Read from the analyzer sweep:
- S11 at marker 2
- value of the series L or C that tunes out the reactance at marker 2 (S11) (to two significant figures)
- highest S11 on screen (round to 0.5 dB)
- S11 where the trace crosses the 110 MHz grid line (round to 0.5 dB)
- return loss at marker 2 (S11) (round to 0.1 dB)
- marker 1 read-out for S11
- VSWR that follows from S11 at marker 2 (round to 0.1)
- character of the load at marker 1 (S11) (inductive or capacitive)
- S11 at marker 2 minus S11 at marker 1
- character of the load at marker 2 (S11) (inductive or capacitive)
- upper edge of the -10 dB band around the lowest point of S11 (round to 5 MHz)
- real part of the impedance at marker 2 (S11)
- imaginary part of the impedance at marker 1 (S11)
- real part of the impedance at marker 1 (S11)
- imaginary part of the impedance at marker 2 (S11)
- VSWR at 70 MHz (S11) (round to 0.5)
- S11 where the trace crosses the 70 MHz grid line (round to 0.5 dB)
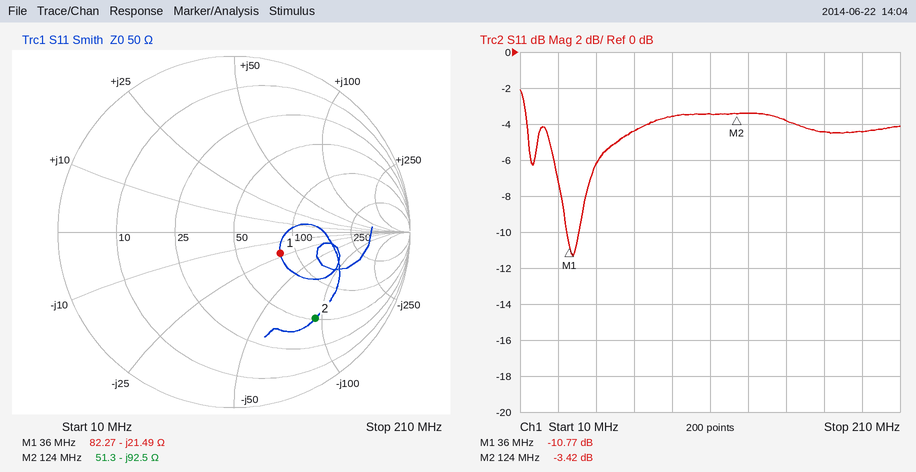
-3.42 dB
120 nH
-2.0 dB
-3.5 dB
3.4 dB
-10.77 dB
5.1
capacitive
7.35 dB
capacitive
40 MHz
51.3 Ω
-21.49 Ω
82.27 Ω
-92.5 Ω
4.0
-4.5 dB
